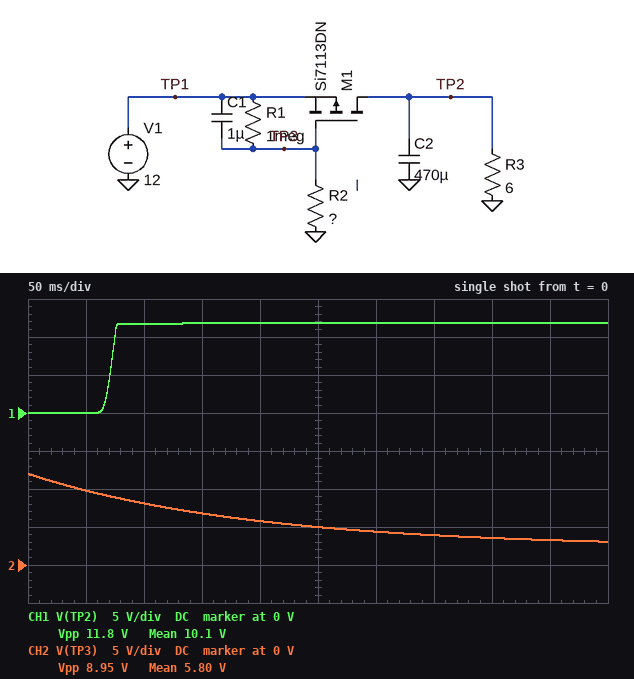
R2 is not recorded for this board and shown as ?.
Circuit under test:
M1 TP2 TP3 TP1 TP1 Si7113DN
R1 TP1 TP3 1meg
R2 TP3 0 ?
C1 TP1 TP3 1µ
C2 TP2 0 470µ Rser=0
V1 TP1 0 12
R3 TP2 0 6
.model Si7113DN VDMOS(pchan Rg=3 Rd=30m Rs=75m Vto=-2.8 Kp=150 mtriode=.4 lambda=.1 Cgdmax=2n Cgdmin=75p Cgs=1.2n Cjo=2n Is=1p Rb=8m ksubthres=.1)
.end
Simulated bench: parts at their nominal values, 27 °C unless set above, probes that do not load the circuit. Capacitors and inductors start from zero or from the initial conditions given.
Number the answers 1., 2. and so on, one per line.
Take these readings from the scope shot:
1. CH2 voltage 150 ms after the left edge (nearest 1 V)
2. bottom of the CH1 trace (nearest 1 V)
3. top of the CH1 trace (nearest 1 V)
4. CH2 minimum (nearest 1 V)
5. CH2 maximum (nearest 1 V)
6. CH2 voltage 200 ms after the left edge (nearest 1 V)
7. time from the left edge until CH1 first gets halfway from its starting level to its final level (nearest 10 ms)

1. 7 V
2. 0 V
3. 12 V
4. 3 V
5. 12 V
6. 6 V
7. 70 ms
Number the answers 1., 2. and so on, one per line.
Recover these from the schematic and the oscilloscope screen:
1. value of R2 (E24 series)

1. 240 kΩ
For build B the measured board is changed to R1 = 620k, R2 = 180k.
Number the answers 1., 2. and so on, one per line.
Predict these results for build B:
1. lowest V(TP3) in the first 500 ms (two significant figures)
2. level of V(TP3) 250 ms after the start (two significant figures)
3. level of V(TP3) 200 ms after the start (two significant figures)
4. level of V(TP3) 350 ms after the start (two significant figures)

1. 3.0 V
2. 4.3 V
3. 4.9 V
4. 3.5 V
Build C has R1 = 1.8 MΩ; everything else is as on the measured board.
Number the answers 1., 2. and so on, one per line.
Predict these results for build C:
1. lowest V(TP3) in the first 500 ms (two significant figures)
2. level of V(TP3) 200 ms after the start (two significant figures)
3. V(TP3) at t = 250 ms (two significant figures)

1. 2.4 V
2. 5.5 V
3. 4.7 V
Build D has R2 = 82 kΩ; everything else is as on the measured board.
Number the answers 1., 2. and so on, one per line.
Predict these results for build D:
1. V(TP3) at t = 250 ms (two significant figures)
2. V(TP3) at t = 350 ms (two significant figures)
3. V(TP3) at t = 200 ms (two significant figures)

1. 1.3 V
2. 1.0 V
3. 1.7 V
